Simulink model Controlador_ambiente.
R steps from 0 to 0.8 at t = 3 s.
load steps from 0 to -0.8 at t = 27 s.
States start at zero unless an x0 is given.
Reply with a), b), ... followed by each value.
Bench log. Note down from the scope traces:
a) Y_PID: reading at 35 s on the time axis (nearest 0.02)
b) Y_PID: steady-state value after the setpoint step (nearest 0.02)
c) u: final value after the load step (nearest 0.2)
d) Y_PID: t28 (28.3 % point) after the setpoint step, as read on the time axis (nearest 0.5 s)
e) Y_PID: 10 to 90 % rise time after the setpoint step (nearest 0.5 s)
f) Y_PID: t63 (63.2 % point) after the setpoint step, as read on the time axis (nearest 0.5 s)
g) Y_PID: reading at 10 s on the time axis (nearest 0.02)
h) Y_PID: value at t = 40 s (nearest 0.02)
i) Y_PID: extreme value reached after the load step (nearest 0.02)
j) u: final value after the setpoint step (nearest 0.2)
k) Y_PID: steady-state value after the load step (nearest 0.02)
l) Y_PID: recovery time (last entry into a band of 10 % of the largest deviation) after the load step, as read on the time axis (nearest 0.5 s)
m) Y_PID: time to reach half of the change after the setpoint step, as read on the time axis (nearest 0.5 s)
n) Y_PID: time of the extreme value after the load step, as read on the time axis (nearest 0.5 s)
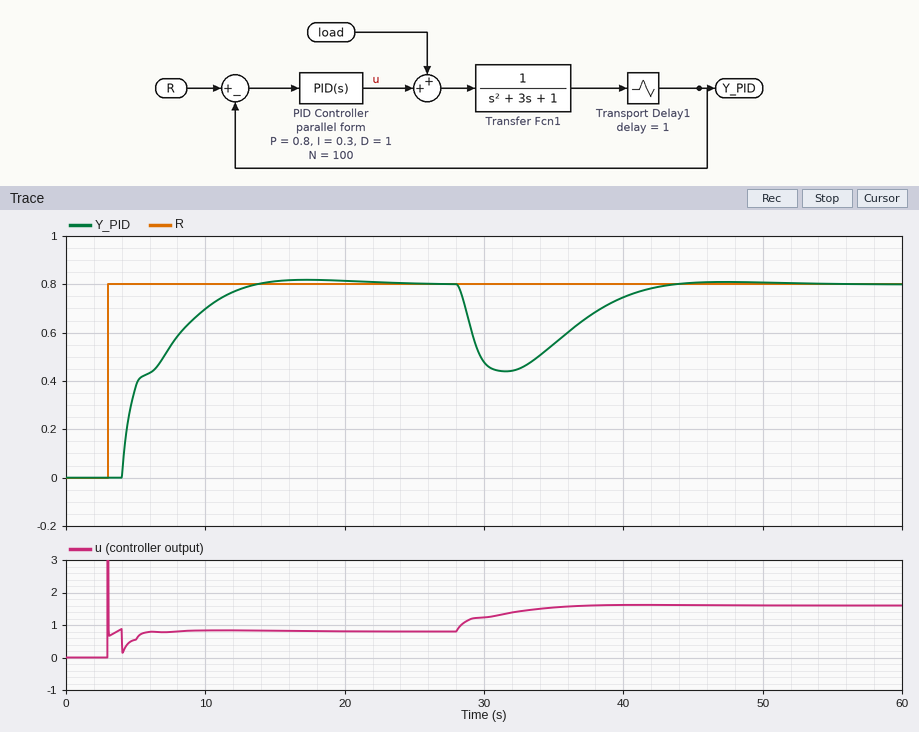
a) 0.56
b) 0.80
c) 1.6
d) 4.5 s
e) 6.5 s
f) 7.0 s
g) 0.70
h) 0.74
i) 0.44
j) 0.8
k) 0.80
l) 41.0 s
m) 5.0 s
n) 31.5 s
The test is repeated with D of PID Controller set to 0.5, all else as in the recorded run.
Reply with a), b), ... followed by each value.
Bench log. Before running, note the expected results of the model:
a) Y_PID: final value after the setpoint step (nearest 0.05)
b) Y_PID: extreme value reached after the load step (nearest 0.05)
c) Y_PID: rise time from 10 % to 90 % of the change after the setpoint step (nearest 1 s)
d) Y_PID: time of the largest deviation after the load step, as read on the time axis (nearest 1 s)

a) 0.80
b) 0.40
c) 5 s
d) 31 s
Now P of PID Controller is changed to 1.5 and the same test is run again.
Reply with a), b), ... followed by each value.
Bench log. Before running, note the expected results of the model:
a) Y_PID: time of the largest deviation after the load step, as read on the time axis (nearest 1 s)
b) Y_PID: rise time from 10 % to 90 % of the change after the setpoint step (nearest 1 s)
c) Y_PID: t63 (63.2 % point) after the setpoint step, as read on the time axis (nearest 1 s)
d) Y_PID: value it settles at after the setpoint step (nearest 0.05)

a) 30 s
b) 7 s
c) 5 s
d) 0.80
